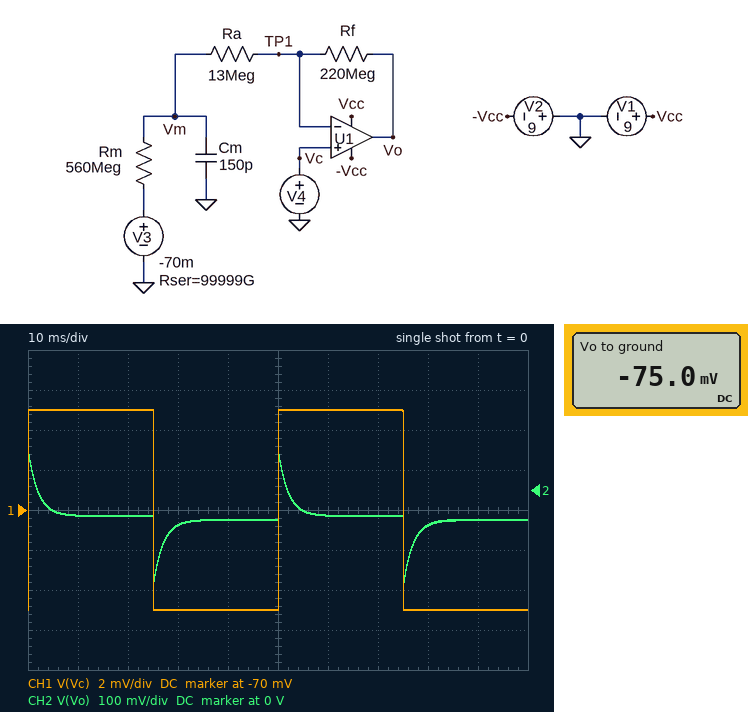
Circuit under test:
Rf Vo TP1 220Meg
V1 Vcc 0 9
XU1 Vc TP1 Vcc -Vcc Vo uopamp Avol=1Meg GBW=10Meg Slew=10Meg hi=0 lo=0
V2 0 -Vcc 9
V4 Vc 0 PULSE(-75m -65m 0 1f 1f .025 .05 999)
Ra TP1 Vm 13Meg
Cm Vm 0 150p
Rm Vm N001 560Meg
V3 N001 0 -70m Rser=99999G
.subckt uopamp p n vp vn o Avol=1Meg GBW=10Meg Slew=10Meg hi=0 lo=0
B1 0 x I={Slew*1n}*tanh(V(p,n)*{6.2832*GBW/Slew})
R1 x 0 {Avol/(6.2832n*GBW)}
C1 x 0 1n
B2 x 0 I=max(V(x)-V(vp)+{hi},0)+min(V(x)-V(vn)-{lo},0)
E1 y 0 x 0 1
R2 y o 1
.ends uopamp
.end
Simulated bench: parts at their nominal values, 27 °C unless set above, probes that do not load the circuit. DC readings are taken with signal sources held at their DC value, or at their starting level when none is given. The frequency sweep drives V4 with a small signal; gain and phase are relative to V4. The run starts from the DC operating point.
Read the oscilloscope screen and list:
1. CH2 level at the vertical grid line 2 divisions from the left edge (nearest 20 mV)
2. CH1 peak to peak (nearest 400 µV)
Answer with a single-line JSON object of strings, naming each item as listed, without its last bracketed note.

{"CH2 level at the vertical grid line 2 divisions from the left edge": "-60 mV", "CH1 peak to peak": "10.0 mV"}
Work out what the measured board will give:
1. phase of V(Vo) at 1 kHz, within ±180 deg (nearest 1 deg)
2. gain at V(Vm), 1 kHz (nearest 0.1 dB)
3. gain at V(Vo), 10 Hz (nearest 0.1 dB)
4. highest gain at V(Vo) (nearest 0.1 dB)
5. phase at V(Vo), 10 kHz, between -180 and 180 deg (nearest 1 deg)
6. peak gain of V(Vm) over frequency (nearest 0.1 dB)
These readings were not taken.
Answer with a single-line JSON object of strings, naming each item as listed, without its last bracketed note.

{"phase of V(Vo) at 1 kHz, within ±180 deg": "4 deg", "gain at V(Vm), 1 kHz": "-21.8 dB", "gain at V(Vo), 10 Hz": "7.6 dB", "highest gain at V(Vo)": "25.1 dB", "phase at V(Vo), 10 kHz, between -180 and 180 deg": "-1 deg", "peak gain of V(Vm) over frequency": "0 dB"}
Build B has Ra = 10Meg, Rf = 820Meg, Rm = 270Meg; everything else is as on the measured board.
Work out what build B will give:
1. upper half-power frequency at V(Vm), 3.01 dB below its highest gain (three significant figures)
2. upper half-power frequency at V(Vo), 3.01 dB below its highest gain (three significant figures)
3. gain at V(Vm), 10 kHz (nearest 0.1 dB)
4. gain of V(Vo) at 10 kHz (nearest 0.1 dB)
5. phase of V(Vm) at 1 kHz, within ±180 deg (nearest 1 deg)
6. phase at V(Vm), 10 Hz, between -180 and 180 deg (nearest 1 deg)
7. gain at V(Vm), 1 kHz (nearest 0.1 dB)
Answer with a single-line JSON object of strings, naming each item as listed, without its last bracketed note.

{"upper half-power frequency at V(Vm), 3.01 dB below its highest gain": "106 Hz", "upper half-power frequency at V(Vo), 3.01 dB below its highest gain": "121 kHz", "gain at V(Vm), 10 kHz": "-39.5 dB", "gain of V(Vo) at 10 kHz": "38.4 dB", "phase of V(Vm) at 1 kHz, within ±180 deg": "-84 deg", "phase at V(Vm), 10 Hz, between -180 and 180 deg": "-5 deg", "gain at V(Vm), 1 kHz": "-19.5 dB"}
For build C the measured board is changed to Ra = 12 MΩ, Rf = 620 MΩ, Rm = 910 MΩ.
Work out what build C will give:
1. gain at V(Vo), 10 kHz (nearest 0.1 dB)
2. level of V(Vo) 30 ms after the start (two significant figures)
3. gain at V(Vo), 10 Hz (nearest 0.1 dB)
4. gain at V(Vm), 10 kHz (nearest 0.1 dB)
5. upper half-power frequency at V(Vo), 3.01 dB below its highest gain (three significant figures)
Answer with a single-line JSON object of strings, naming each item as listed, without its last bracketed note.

{"gain at V(Vo), 10 kHz": "34.4 dB", "level of V(Vo) 30 ms after the start": "-110 mV", "gain at V(Vo), 10 Hz": "15.6 dB", "gain at V(Vm), 10 kHz": "-41.1 dB", "upper half-power frequency at V(Vo), 3.01 dB below its highest gain": "190 kHz"}
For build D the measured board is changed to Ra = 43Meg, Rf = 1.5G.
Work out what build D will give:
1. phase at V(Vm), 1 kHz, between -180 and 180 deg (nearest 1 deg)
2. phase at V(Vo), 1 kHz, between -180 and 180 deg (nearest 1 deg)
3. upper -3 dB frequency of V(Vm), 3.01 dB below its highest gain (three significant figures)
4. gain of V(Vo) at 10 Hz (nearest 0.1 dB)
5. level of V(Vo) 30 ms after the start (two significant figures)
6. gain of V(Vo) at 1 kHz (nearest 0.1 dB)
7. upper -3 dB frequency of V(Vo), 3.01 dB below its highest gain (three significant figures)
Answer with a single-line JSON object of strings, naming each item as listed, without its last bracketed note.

{"phase at V(Vm), 1 kHz, between -180 and 180 deg": "-89 deg", "phase at V(Vo), 1 kHz, between -180 and 180 deg": "1 deg", "upper -3 dB frequency of V(Vm), 3.01 dB below its highest gain": "24.7 Hz", "gain of V(Vo) at 10 Hz": "22.6 dB", "level of V(Vo) 30 ms after the start": "-230 mV", "gain of V(Vo) at 1 kHz": "31.1 dB", "upper -3 dB frequency of V(Vo), 3.01 dB below its highest gain": "279 kHz"}
